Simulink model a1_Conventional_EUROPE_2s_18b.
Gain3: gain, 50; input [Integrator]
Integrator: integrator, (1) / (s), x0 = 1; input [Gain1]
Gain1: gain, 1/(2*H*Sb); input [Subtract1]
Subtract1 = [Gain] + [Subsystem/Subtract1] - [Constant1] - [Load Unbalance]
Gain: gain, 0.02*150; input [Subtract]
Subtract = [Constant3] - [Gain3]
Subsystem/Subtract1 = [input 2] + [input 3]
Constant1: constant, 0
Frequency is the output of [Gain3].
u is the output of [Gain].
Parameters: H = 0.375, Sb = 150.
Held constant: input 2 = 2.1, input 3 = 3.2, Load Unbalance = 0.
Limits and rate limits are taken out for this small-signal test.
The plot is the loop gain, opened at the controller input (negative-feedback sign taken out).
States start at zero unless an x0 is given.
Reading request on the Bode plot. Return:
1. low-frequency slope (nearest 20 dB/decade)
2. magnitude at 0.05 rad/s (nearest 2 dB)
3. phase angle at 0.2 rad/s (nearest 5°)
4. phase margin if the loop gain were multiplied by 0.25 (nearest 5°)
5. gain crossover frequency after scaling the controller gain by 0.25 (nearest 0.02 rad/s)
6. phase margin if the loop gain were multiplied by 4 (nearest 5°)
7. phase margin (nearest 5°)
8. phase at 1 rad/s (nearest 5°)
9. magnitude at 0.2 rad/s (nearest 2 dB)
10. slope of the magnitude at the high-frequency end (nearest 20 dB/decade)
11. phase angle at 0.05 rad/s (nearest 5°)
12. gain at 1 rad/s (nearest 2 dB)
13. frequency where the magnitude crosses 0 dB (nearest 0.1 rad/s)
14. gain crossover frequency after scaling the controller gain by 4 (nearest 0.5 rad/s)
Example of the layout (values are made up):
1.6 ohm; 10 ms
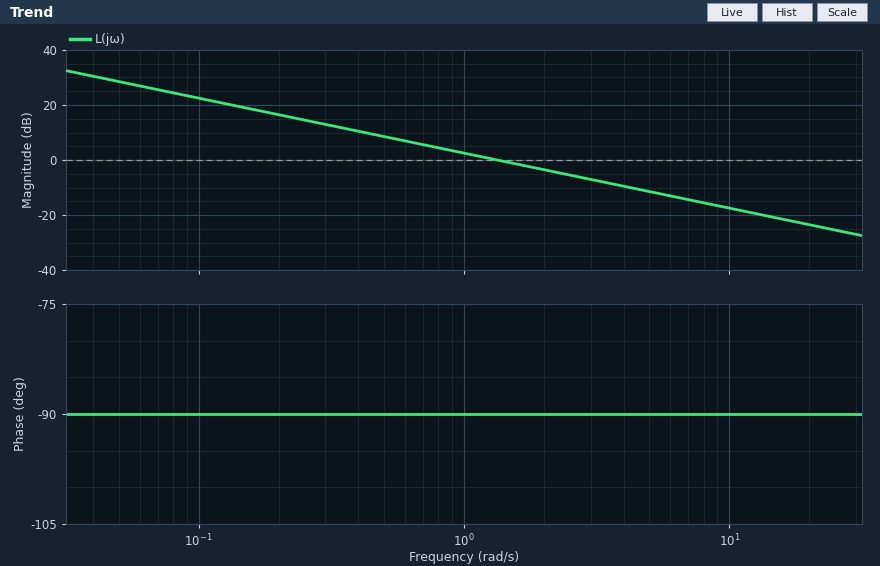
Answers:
-20 dB/decade; 28 dB; -90°; 90°; 0.34 rad/s; 90°; 90°; -90°; 16 dB; -20 dB/decade; -90°; 2 dB; 1.3 rad/s; 5.5 rad/s
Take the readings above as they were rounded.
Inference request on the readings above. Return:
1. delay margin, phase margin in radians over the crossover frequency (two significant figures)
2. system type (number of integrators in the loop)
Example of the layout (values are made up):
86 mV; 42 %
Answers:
1.2 s; 1
